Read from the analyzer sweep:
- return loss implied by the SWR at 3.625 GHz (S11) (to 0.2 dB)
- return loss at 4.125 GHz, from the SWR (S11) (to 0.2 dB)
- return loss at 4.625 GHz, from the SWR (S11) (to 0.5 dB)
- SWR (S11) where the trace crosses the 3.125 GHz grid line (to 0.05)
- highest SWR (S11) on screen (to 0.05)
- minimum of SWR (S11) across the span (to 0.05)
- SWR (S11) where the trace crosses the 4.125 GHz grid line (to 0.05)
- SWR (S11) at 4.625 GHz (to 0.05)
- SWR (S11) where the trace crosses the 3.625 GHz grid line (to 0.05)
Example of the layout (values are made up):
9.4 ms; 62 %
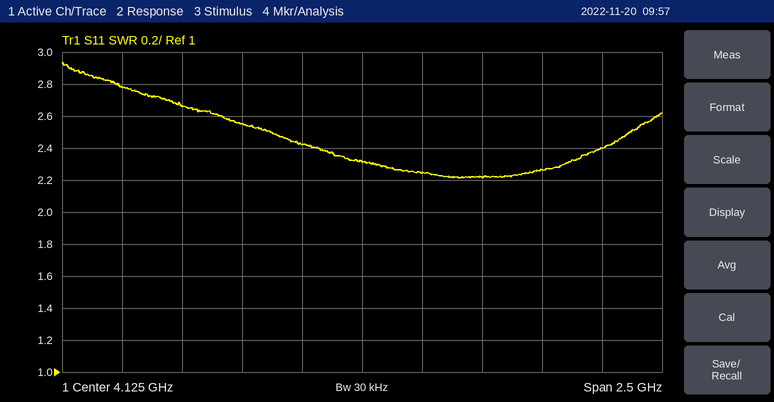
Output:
7.2 dB; 8.0 dB; 8.5 dB; 2.80; 2.95; 2.20; 2.30; 2.20; 2.55
